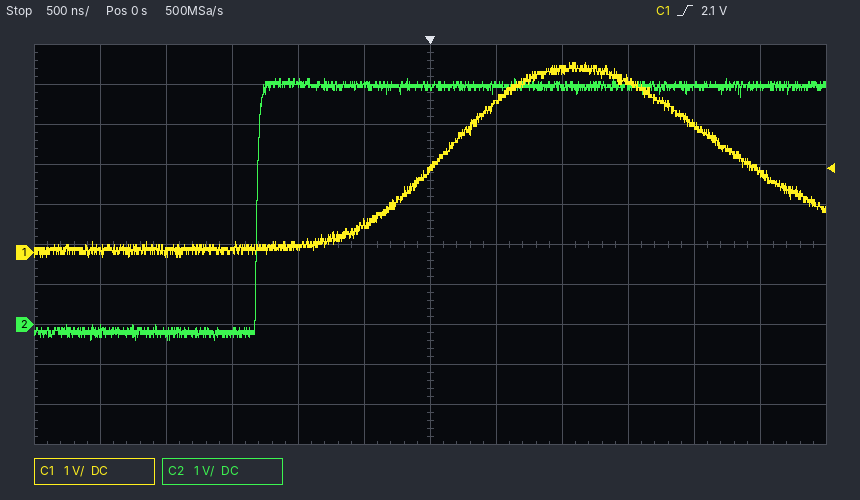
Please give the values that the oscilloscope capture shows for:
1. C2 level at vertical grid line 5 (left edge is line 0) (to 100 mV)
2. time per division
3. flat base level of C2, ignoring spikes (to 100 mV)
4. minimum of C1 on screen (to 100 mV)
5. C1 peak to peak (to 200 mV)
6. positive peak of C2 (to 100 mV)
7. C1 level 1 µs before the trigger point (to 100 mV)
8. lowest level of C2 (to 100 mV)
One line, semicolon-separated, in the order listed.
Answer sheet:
6.0 V; 500 ns; -200 mV; -100 mV; 4.8 V; 6.2 V; 100 mV; -400 mV
